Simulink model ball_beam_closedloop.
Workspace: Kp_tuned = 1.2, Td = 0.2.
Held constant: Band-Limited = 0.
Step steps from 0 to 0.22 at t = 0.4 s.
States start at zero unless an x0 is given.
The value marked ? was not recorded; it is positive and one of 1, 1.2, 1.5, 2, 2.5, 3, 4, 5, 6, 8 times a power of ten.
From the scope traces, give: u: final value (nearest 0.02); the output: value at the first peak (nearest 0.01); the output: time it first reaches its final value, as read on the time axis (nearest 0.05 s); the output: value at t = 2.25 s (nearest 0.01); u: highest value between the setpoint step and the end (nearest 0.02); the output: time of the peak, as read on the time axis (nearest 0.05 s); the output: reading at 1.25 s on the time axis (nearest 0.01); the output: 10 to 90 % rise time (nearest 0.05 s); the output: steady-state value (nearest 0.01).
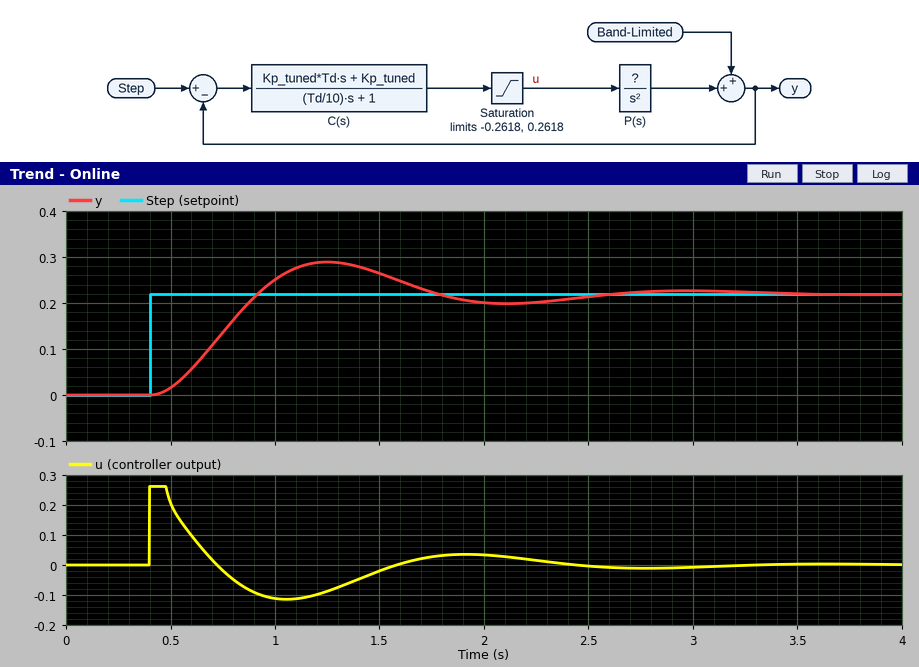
0.00
0.29
0.90 s
0.20
0.26
1.25 s
0.29
0.35 s
0.22
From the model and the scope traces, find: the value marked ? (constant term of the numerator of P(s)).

12
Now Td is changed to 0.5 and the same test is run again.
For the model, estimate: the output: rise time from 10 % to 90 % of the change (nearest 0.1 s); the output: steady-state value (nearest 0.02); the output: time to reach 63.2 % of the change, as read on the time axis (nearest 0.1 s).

0.6 s
0.22
0.8 s
